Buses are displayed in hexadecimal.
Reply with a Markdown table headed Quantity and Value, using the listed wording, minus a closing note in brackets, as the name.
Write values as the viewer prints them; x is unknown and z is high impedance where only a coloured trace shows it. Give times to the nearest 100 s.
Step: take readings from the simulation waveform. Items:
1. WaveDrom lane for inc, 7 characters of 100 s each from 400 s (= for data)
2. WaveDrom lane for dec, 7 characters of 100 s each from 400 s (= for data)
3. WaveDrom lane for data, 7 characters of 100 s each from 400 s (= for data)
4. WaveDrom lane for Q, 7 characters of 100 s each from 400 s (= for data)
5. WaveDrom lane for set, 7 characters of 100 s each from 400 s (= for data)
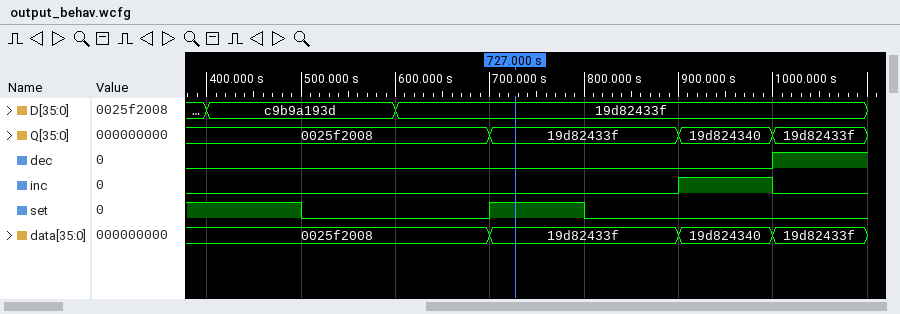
| Quantity | Value |
|---|---|
| WaveDrom lane for inc, 7 characters of 100 s each from 400 s | {name: 'inc', wave: '0....10'} |
| WaveDrom lane for dec, 7 characters of 100 s each from 400 s | {name: 'dec', wave: '0.....1'} |
| WaveDrom lane for data, 7 characters of 100 s each from 400 s | {name: 'data', wave: '=..=.==', data: '0025f2008 19d82433f 19d824340 19d82433f'} |
| WaveDrom lane for Q, 7 characters of 100 s each from 400 s | {name: 'Q', wave: '=..=.==', data: '0025f2008 19d82433f 19d824340 19d82433f'} |
| WaveDrom lane for set, 7 characters of 100 s each from 400 s | {name: 'set', wave: '10.10..'} |
